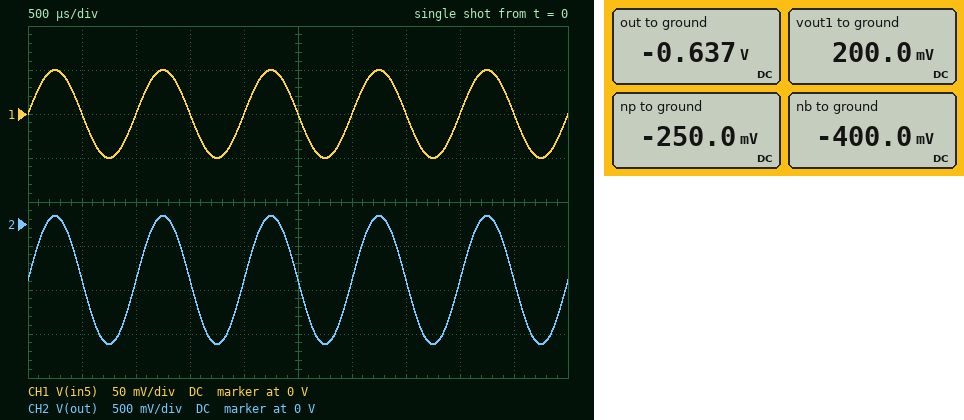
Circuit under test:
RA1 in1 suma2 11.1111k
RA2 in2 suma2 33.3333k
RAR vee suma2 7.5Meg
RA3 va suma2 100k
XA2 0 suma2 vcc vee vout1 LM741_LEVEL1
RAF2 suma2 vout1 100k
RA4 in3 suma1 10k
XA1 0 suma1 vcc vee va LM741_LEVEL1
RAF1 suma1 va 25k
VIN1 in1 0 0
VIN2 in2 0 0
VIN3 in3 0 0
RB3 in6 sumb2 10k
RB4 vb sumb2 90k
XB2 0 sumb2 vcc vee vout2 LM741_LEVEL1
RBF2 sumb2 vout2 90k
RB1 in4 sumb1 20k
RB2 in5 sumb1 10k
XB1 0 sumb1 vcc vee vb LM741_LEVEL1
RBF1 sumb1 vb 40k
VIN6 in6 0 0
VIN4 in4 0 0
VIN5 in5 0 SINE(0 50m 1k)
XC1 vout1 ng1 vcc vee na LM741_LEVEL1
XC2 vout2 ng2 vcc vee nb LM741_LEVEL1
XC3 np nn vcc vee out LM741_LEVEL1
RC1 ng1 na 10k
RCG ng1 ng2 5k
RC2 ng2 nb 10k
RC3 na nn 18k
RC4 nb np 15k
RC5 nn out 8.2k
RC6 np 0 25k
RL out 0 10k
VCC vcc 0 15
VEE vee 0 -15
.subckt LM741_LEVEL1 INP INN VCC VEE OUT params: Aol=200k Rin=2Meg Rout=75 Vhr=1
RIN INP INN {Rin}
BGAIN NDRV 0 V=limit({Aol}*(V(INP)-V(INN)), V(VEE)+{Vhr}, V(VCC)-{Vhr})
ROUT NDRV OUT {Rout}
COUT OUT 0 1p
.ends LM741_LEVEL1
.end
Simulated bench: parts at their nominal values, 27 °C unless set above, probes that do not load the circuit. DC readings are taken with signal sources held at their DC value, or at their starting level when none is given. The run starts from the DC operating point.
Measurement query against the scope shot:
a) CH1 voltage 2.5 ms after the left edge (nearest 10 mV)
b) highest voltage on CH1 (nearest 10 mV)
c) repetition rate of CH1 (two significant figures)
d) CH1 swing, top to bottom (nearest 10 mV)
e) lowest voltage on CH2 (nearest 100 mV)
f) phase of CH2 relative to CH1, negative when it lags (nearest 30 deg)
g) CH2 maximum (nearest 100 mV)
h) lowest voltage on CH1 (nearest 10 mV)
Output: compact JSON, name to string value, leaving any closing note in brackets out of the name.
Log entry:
{"CH1 voltage 2.5 ms after the left edge": "0 V", "highest voltage on CH1": "50 mV", "repetition rate of CH1": "1.0 kHz", "CH1 swing, top to bottom": "100 mV", "lowest voltage on CH2": "-1.4 V", "phase of CH2 relative to CH1, negative when it lags": "0 deg", "CH2 maximum": "100 mV", "lowest voltage on CH1": "-50 mV"}
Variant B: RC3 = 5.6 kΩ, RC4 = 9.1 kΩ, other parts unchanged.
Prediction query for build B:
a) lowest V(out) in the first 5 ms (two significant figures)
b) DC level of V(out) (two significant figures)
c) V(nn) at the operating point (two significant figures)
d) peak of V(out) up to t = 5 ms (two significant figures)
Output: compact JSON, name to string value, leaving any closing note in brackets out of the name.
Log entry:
{"lowest V(out) in the first 5 ms": "-3.3 V", "DC level of V(out)": "-1.6 V", "V(nn) at the operating point": "-290 mV", "peak of V(out) up to t = 5 ms": "68 mV"}
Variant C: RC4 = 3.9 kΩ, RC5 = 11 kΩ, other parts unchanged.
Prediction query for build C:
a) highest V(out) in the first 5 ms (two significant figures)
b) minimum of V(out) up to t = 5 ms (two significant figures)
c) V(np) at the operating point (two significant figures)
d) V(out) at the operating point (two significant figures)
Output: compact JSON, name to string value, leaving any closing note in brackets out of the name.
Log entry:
{"highest V(out) in the first 5 ms": "160 mV", "minimum of V(out) up to t = 5 ms": "-2.0 V", "V(np) at the operating point": "-350 mV", "V(out) at the operating point": "-920 mV"}
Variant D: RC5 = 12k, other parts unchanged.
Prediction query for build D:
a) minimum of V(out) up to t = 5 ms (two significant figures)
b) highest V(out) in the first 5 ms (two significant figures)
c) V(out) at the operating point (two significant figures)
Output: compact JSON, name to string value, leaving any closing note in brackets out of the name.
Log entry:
{"minimum of V(out) up to t = 5 ms": "-1.7 V", "highest V(out) in the first 5 ms": "75 mV", "V(out) at the operating point": "-820 mV"}
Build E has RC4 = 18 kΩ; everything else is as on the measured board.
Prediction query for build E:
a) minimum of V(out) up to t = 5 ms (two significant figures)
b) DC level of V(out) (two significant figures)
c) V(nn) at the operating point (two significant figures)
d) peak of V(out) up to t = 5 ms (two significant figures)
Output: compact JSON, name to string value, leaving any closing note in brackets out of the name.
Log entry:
{"minimum of V(out) up to t = 5 ms": "-1.3 V", "DC level of V(out)": "-610 mV", "V(nn) at the operating point": "-230 mV", "peak of V(out) up to t = 5 ms": "78 mV"}
